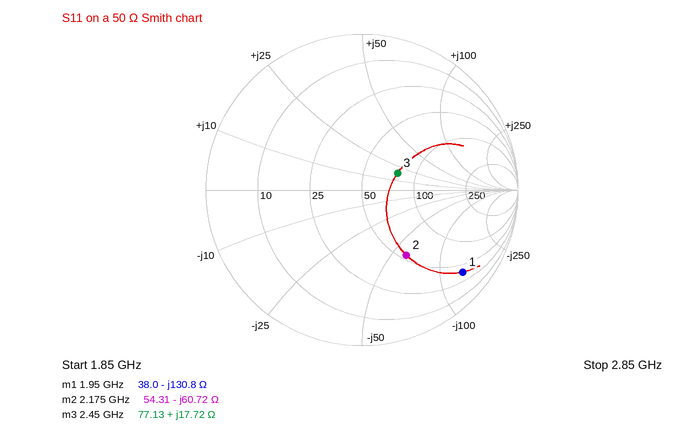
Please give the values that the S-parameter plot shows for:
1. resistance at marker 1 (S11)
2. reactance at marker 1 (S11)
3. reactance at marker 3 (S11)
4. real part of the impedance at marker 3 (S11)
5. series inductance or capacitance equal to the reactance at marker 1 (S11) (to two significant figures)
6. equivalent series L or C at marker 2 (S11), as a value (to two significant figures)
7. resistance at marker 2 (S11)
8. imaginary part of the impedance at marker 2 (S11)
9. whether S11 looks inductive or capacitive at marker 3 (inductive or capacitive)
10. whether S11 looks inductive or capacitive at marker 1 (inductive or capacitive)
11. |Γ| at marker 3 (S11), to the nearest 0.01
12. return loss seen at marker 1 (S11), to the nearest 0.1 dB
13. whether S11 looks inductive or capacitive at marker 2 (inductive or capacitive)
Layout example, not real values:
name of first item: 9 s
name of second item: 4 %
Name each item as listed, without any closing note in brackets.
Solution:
resistance at marker 1: 38.0 Ω
reactance at marker 1: -130.8 Ω
reactance at marker 3: +17.72 Ω
real part of the impedance at marker 3: 77.13 Ω
series inductance or capacitance equal to the reactance at marker 1 (S11): 620 fF
equivalent series L or C at marker 2 (S11), as a value: 1.2 pF
resistance at marker 2: 54.31 Ω
imaginary part of the impedance at marker 2: -60.72 Ω
whether S11 looks inductive or capacitive at marker 3: inductive
whether S11 looks inductive or capacitive at marker 1: capacitive
|Γ| at marker 3 (S11), to the nearest 0.01: 0.25
return loss seen at marker 1 (S11), to the nearest 0.1 dB: 1.6 dB
whether S11 looks inductive or capacitive at marker 2: capacitive
